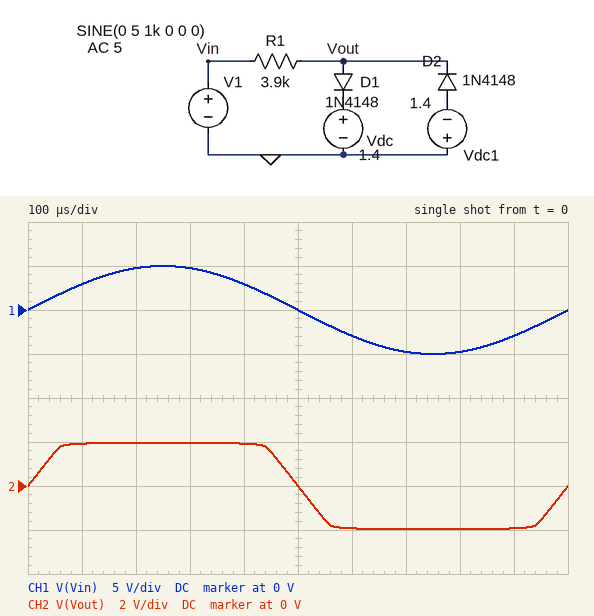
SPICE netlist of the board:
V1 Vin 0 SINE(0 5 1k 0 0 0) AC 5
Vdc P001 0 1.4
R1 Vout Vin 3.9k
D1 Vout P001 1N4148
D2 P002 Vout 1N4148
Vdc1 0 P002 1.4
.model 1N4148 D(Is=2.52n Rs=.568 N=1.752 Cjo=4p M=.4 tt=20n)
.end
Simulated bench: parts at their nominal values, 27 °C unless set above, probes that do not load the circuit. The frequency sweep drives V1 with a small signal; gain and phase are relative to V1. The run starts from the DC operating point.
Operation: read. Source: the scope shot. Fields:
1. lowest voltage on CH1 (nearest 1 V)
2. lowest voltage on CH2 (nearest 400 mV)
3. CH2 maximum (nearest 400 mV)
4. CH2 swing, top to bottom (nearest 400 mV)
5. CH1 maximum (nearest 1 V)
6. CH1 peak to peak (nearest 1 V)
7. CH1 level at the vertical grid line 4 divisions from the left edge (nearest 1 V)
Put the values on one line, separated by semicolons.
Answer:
-5 V; -2.0 V; 2.0 V; 4.0 V; 5 V; 10 V; 3 V
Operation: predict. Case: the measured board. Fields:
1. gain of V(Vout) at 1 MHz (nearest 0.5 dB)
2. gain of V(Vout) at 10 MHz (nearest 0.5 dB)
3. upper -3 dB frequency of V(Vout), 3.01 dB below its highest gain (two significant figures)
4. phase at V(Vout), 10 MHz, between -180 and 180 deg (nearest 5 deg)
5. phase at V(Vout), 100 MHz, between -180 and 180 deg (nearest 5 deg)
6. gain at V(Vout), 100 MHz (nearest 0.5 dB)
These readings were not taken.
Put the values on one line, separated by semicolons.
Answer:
0 dB; -4.5 dB; 7.2 MHz; -55 deg; -85 deg; -23.0 dB
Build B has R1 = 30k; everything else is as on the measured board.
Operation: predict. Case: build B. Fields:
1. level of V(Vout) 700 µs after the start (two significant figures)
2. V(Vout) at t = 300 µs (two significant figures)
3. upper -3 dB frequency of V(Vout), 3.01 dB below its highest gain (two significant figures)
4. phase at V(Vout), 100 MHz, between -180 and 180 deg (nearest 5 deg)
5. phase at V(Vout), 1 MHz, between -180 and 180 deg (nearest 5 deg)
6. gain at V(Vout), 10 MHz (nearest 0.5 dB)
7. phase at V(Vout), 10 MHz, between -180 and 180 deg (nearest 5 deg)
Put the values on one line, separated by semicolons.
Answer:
-1.9 V; 1.9 V; 940 kHz; -90 deg; -45 deg; -20.5 dB; -85 deg
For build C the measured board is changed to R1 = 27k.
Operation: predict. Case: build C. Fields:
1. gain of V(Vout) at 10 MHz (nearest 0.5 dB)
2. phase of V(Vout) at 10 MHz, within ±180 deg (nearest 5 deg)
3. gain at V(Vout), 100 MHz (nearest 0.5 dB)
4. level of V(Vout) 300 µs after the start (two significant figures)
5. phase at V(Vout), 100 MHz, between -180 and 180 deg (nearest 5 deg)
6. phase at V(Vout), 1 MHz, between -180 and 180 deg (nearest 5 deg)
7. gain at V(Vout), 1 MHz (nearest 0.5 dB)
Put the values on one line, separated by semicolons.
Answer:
-19.5 dB; -85 deg; -39.5 dB; 1.9 V; -90 deg; -45 deg; -3.0 dB
